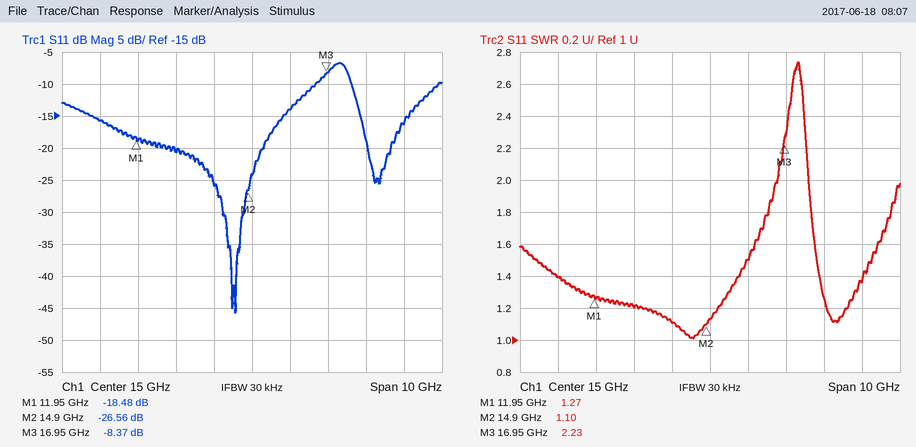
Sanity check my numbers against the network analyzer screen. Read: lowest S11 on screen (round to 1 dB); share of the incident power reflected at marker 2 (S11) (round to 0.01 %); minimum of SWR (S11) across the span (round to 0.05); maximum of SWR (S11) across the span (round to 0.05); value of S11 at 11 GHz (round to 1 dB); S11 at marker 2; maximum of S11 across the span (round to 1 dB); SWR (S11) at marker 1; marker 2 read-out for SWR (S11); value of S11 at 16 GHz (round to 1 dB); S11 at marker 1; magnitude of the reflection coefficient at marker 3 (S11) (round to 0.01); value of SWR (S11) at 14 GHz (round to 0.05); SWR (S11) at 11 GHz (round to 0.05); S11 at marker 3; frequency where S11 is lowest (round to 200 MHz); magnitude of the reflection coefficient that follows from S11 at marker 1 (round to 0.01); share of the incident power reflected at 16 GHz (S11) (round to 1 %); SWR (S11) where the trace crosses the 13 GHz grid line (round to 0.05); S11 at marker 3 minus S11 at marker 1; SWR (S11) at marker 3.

-46 dB
0.22 %
1.00
2.75
-16 dB
-26.56 dB
-7 dB
1.27
1.10
-14 dB
-18.48 dB
0.38
1.10
1.40
-8.37 dB
14.6 GHz
0.12
4 %
1.20
10.11 dB
2.23
